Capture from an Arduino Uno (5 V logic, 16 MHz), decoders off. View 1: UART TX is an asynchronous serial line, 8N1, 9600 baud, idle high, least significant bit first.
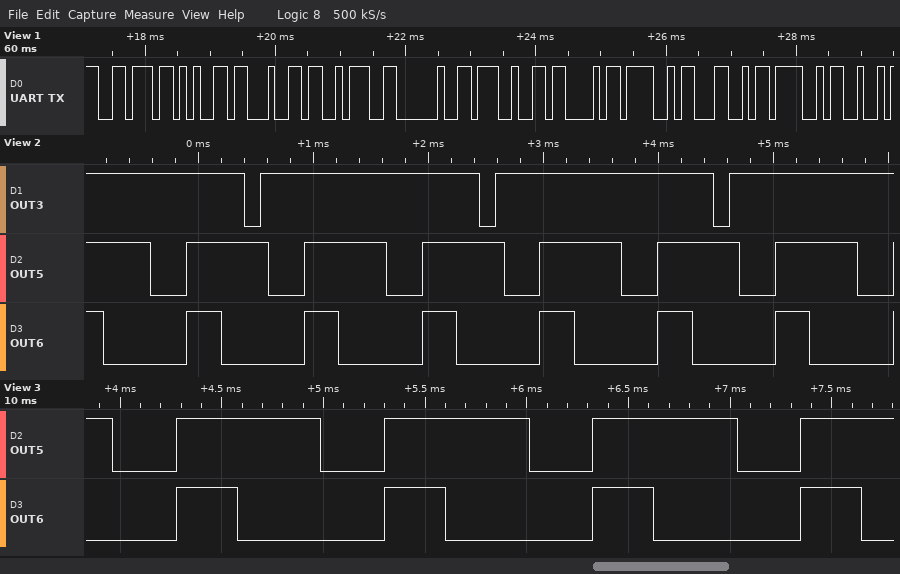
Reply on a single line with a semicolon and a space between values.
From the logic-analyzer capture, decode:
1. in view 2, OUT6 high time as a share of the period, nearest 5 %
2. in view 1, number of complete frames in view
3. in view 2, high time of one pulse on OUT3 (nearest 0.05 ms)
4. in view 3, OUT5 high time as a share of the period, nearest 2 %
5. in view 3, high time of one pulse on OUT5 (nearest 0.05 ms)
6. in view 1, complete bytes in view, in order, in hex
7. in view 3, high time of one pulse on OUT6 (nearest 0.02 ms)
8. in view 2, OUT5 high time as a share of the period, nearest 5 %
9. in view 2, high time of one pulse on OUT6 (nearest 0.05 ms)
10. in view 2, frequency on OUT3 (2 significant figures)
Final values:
30 %; 10; 1.90 ms; 70 %; 0.70 ms; 76 65 64 3A 20 27 43 4F 4C 4F; 0.30 ms; 70 %; 0.30 ms; 490 Hz
